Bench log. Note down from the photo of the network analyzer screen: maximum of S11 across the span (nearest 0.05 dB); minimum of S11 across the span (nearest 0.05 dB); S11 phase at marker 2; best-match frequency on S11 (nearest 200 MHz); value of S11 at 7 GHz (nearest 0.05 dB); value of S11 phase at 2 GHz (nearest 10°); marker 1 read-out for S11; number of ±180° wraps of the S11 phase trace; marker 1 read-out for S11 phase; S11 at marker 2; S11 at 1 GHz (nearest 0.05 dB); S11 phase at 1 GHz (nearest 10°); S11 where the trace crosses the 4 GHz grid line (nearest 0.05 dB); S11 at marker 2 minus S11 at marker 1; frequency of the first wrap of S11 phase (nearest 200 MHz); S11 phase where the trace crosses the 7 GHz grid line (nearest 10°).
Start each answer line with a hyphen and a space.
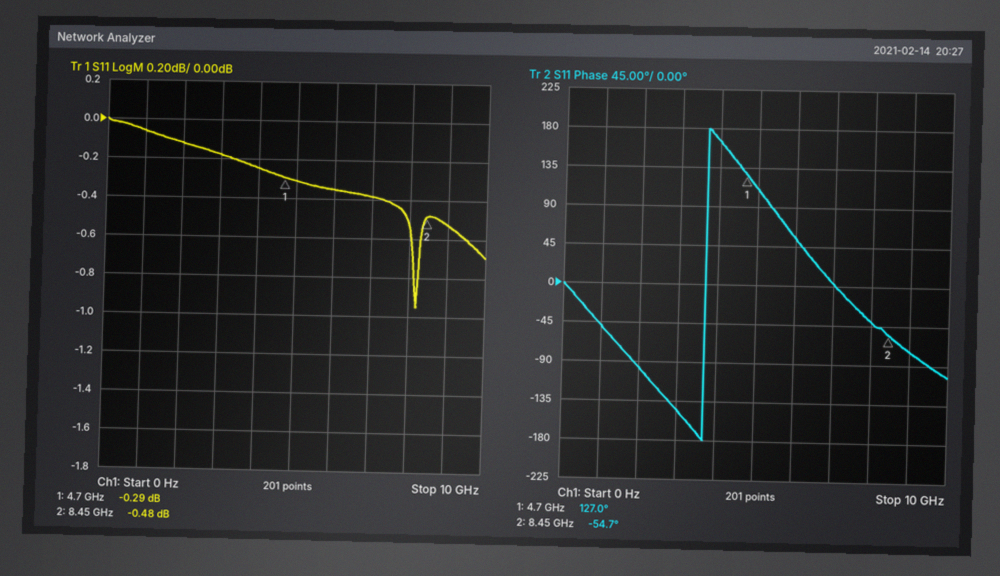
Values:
- 0.00 dB
- -0.95 dB
- -54.7°
- 8.2 GHz
- -0.40 dB
- -100°
- -0.29 dB
- 1
- 127.0°
- -0.48 dB
- -0.05 dB
- -50°
- -0.25 dB
- -0.19 dB
- 3.8 GHz
- 0°
